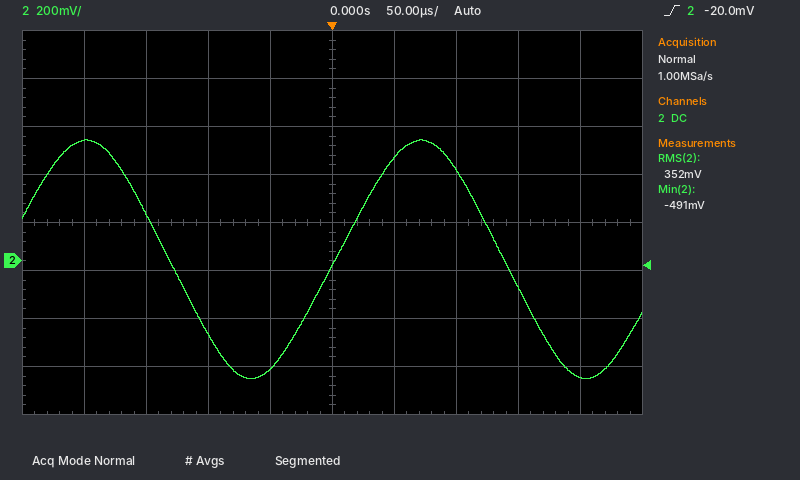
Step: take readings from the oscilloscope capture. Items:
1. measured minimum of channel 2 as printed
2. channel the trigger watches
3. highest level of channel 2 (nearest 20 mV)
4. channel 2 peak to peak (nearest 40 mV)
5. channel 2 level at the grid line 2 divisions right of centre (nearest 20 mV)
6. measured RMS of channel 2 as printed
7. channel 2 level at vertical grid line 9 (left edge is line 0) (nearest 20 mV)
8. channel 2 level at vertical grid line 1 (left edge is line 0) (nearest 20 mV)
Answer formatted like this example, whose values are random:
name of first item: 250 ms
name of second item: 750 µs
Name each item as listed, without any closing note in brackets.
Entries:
measured minimum of channel 2 as printed: -491 mV
channel the trigger watches: channel 2
highest level of channel 2: 500 mV
channel 2 peak to peak: 1.00 V
channel 2 level at the grid line 2 divisions right of centre: 380 mV
measured RMS of channel 2 as printed: 352 mV
channel 2 level at vertical grid line 9 (left edge is line 0): -480 mV
channel 2 level at vertical grid line 1 (left edge is line 0): 500 mV
